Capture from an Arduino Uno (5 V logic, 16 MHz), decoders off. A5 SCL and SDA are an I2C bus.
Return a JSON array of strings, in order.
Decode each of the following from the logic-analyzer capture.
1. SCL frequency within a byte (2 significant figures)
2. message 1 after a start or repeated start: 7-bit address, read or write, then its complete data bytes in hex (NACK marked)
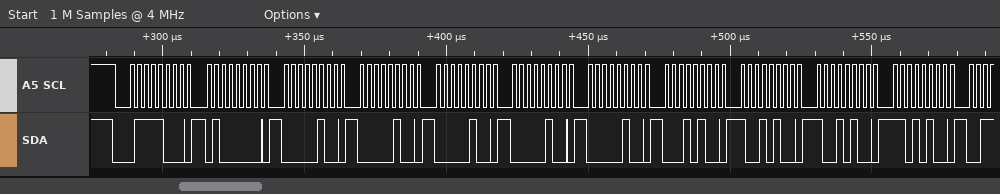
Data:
["400 kHz", "0x3C write: 40 04 04 04 04 04 14 94 94 D4"]
